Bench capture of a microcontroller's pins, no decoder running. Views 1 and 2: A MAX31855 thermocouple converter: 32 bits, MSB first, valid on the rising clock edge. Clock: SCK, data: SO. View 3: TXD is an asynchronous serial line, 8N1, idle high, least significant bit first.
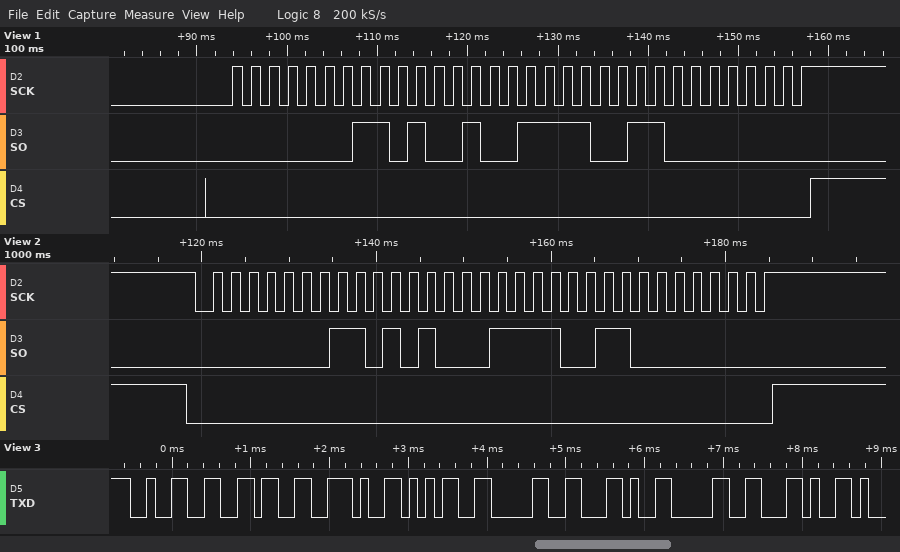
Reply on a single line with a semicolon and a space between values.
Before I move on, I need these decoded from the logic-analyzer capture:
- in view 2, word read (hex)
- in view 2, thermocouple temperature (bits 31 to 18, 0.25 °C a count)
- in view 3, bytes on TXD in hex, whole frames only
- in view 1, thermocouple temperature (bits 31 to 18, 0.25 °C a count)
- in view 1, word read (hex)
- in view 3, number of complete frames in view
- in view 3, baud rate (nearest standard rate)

0x01A8F300; 26.50 °C; 32 36 2E 35 30 2C 30 2C; 26.25 °C; 0x01A4F300; 8; 9600 baud
